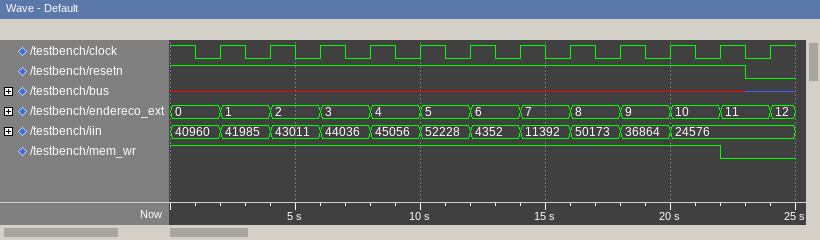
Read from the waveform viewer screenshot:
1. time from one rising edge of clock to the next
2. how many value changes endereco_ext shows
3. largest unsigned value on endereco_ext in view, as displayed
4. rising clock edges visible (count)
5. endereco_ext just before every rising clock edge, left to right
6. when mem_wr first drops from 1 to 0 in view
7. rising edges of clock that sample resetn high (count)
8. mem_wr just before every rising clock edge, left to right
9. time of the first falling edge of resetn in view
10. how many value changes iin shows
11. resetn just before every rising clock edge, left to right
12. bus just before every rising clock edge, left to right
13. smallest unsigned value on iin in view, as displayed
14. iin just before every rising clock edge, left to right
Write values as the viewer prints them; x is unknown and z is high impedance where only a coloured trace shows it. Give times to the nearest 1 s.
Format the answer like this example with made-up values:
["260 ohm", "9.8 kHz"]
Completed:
["2 s", "12", "12", "12", "0, 1, 2, 3, 4, 5, 6, 7, 8, 9, 10, 11", "22 s", "11", "1 1 1 1 1 1 1 1 1 1 1 0", "23 s", "10", "1 1 1 1 1 1 1 1 1 1 1 0", "x, x, x, x, x, x, x, x, x, x, x, z", "4352", "40960, 41985, 43011, 44036, 45056, 52228, 4352, 11392, 50173, 36864, 24576, 24576"]
